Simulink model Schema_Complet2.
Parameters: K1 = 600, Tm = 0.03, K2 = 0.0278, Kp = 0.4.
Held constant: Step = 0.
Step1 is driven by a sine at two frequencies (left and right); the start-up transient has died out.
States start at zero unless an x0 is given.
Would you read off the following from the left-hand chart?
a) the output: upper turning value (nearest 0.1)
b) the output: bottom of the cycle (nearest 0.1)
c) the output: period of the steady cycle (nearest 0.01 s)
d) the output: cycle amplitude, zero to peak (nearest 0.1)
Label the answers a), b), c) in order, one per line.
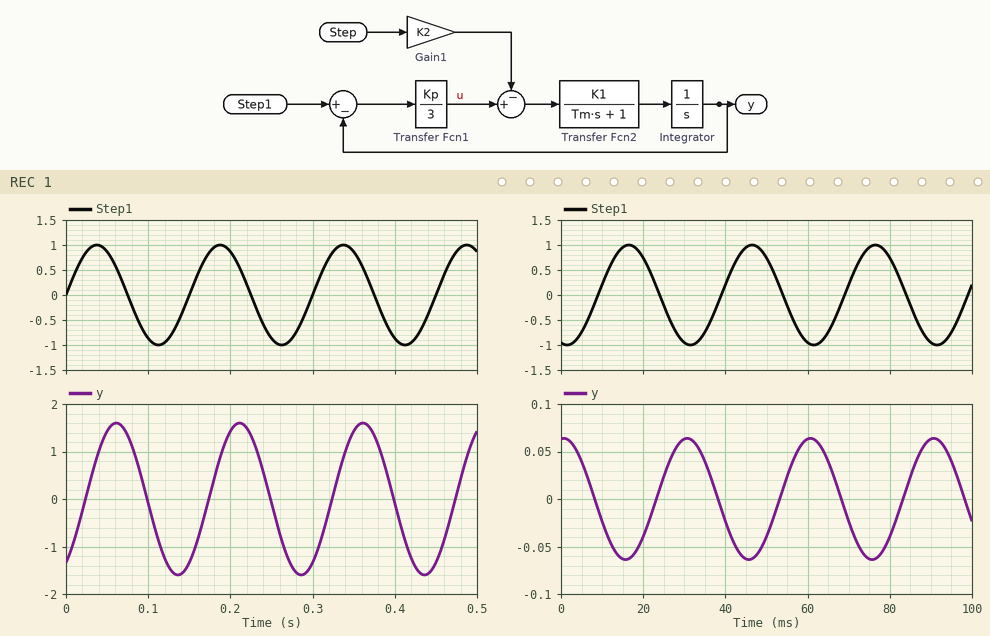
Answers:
a) 1.6
b) -1.6
c) 0.15 s
d) 1.6
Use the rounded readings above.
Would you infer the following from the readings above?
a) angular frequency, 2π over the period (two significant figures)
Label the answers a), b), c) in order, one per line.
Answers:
a) 42 rad/s
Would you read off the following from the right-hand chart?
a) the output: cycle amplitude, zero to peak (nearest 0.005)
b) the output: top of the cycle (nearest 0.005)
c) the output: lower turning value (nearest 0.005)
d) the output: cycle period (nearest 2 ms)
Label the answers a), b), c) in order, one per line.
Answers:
a) 0.065
b) 0.065
c) -0.065
d) 30 ms
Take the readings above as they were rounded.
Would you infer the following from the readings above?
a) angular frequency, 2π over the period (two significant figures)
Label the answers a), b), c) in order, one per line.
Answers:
a) 0.21 rad/ms
